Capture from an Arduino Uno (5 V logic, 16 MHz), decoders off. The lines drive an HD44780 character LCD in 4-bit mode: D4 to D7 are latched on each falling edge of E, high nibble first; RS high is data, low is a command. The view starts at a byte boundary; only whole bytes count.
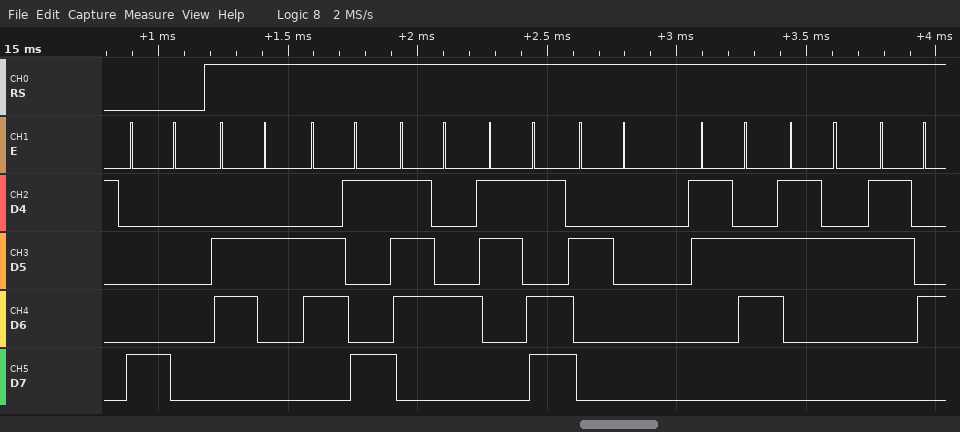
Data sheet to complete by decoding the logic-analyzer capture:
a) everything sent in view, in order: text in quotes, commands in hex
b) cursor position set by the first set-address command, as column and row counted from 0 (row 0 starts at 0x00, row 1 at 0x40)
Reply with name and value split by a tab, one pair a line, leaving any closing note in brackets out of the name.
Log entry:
everything sent in view, in order: text in quotes, commands in hex	0x80 "bit= 624"
cursor position set by the first set-address command, as column and row counted from 0	column 0, row 0
